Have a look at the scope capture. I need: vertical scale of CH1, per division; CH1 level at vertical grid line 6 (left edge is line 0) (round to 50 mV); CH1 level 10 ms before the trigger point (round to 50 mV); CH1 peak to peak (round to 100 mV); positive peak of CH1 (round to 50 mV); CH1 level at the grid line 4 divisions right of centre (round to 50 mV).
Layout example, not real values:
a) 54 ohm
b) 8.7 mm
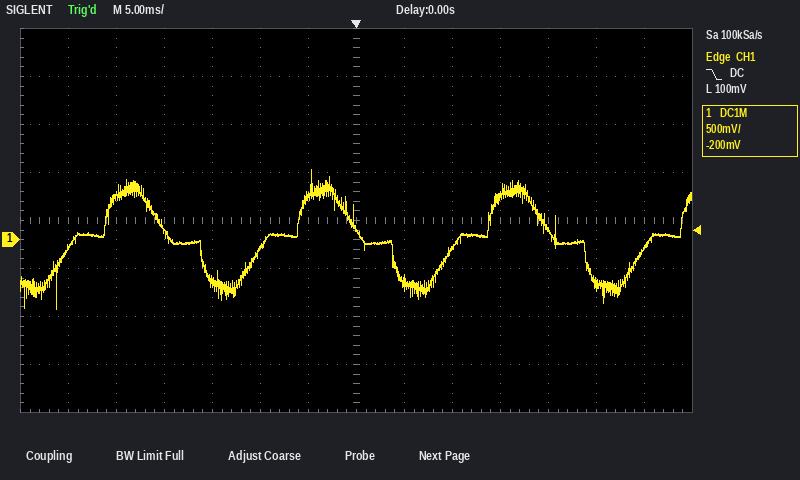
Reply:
a) 500 mV
b) 450 mV
c) -100 mV
d) 1.50 V
e) 750 mV
f) 100 mV
